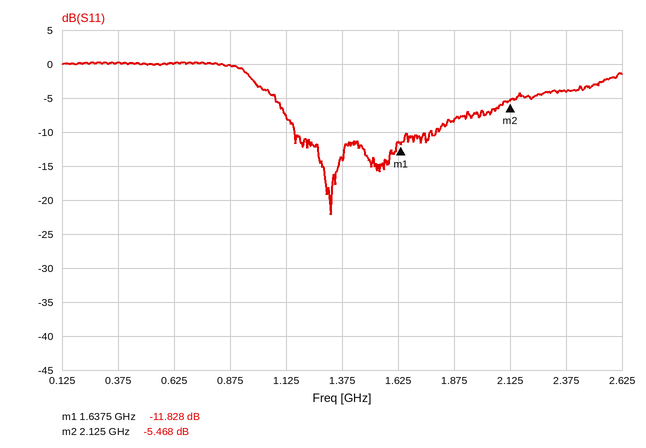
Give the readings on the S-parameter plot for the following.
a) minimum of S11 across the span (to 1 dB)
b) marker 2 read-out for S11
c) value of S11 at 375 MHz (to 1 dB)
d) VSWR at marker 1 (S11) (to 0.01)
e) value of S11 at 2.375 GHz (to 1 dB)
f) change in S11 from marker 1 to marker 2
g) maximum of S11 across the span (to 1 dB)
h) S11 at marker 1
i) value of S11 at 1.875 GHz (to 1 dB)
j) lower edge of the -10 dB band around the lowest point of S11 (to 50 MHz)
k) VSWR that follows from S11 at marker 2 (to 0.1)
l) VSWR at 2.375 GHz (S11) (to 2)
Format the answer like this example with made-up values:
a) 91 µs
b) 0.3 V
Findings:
a) -22 dB
b) -5.468 dB
c) 0 dB
d) 1.69
e) -4 dB
f) 6.360 dB
g) 0 dB
h) -11.828 dB
i) -8 dB
j) 1.15 GHz
k) 3.3
l) 4
